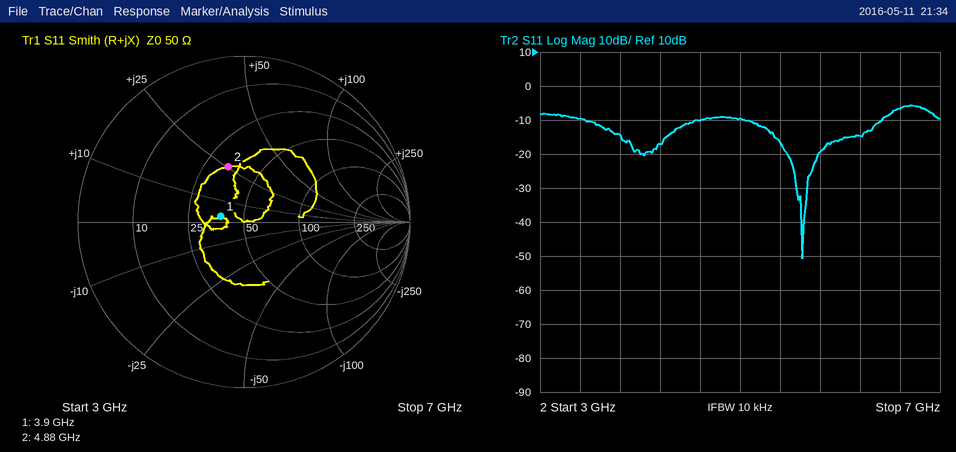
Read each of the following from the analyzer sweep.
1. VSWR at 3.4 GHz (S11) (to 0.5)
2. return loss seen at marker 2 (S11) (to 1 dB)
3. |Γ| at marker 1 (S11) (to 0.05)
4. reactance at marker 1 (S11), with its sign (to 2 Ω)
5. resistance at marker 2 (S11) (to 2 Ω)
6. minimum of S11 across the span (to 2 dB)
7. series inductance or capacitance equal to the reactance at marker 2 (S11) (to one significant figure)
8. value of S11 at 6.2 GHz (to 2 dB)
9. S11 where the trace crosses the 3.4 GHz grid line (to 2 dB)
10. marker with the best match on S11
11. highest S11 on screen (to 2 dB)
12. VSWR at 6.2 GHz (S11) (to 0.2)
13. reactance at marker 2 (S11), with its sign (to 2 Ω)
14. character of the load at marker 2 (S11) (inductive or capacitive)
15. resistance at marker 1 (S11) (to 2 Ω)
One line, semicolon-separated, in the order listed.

2.0; 9 dB; 0.15; +2 Ω; 34 Ω; -50 dB; 800 pH; -14 dB; -10 dB; marker 1; -6 dB; 1.4; +26 Ω; inductive; 38 Ω
